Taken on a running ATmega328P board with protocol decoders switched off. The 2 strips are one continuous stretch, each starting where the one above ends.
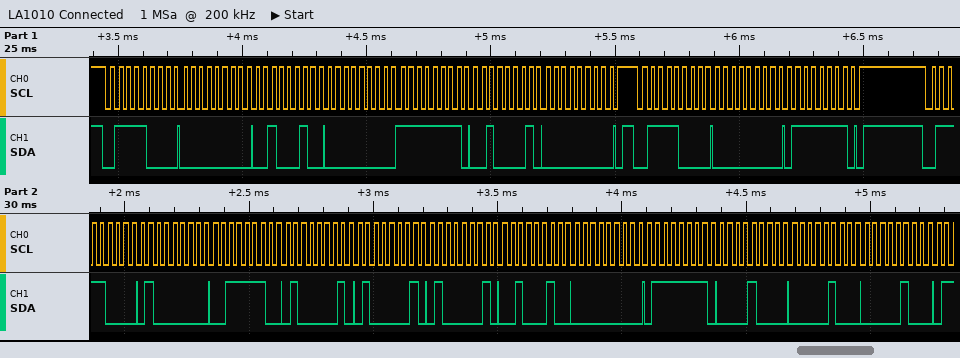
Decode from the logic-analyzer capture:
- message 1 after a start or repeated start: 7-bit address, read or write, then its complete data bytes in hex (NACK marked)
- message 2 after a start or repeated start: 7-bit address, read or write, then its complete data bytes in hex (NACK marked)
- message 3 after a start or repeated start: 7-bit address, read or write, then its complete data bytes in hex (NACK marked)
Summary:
0x3C write: 00 22 00 FF 21 00
0x3C write: 00 7F
0x3C write: 40 3E 41 41 41 22 00 7F 08 04 04
